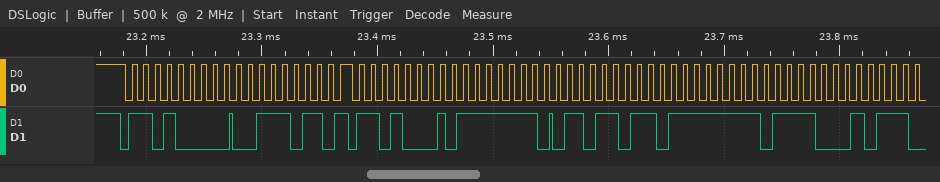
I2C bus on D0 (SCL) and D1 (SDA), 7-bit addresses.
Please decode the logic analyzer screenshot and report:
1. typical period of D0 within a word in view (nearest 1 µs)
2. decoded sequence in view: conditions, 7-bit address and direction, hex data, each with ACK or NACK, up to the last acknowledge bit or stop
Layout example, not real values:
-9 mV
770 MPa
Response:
10 µs
start, address 68 write ACK, 3B ACK, repeated start, address 68 read ACK, FE ACK, DB ACK, FF ACK, F1 ACK
